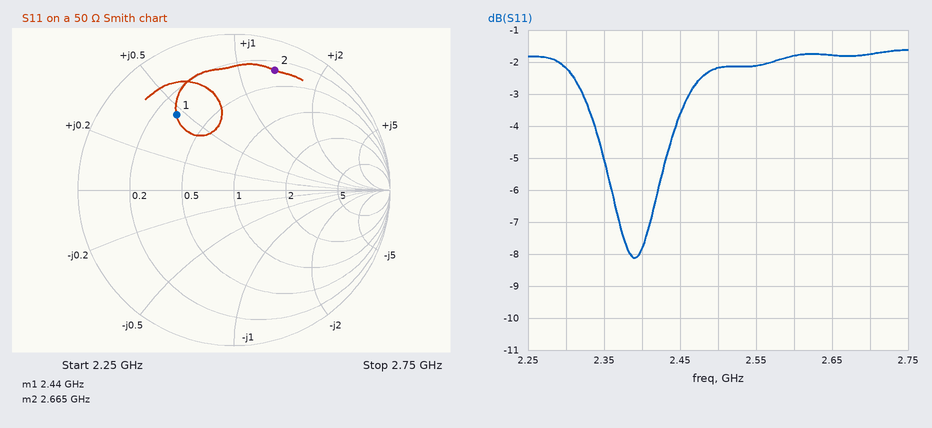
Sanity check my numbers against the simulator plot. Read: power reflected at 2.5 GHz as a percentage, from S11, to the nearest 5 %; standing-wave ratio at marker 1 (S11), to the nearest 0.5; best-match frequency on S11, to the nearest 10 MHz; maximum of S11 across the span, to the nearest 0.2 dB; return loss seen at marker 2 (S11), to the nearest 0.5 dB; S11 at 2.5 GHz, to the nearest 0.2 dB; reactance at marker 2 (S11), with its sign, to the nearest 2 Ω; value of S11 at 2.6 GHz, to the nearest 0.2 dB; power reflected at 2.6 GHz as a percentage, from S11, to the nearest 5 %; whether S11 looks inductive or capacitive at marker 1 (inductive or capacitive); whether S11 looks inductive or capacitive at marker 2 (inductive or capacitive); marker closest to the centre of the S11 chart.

60 %
4.0
2.39 GHz
-1.6 dB
2.0 dB
-2.2 dB
+68 Ω
-1.8 dB
65 %
inductive
inductive
marker 1
